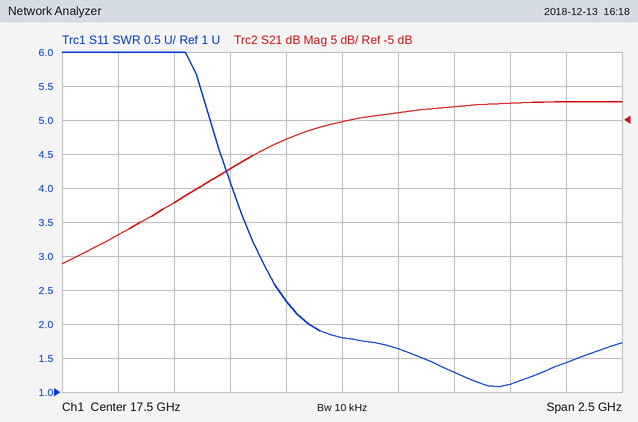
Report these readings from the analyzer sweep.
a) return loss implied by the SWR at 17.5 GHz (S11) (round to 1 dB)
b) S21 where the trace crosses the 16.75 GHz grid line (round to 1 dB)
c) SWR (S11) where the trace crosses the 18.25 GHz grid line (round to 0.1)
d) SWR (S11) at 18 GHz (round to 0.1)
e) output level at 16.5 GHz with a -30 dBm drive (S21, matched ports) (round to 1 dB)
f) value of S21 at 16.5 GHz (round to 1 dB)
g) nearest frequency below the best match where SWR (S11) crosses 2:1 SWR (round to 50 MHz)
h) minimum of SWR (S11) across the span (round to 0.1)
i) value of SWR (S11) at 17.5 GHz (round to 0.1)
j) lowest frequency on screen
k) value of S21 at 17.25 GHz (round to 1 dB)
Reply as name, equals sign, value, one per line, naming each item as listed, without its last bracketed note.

return loss implied by the SWR at 17.5 GHz (S11) = 11 dB
S21 where the trace crosses the 16.75 GHz grid line = -17 dB
SWR (S11) where the trace crosses the 18.25 GHz grid line = 1.1
SWR (S11) at 18 GHz = 1.3
output level at 16.5 GHz with a -30 dBm drive (S21, matched ports) = -52 dBm
value of S21 at 16.5 GHz = -22 dB
nearest frequency below the best match where SWR (S11) crosses 2:1 SWR = 17.35 GHz
minimum of SWR (S11) across the span = 1.1
value of SWR (S11) at 17.5 GHz = 1.8
lowest frequency on screen = 16.25 GHz
value of S21 at 17.25 GHz = -8 dB
